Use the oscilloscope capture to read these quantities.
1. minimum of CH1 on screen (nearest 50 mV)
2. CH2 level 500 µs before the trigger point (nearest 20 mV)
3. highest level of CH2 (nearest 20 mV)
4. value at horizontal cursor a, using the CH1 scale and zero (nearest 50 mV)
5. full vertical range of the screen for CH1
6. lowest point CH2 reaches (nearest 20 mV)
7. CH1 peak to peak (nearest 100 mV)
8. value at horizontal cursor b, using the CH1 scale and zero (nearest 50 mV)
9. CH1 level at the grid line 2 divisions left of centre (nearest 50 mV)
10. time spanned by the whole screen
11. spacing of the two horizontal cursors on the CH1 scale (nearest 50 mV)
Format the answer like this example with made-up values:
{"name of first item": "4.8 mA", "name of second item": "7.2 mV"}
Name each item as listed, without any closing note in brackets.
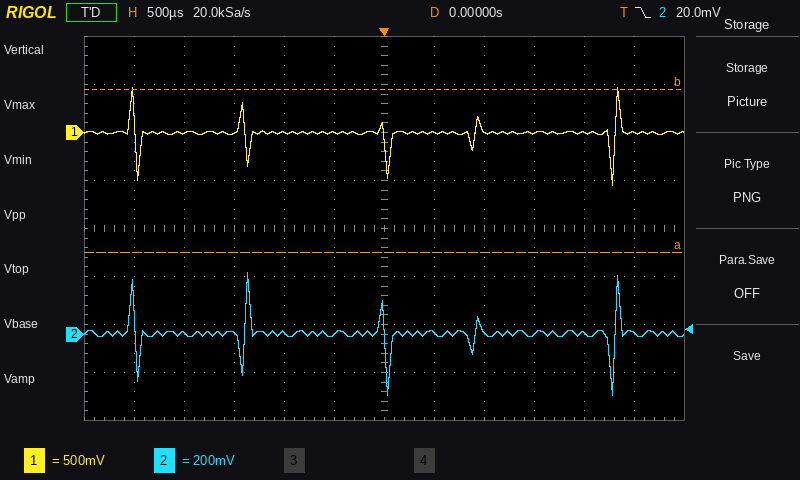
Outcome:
{"minimum of CH1 on screen": "-550 mV", "CH2 level 500 µs before the trigger point": "0 mV", "highest level of CH2": "260 mV", "value at horizontal cursor a, using the CH1 scale and zero": "-1.25 V", "full vertical range of the screen for CH1": "4 V", "lowest point CH2 reaches": "-260 mV", "CH1 peak to peak": "1.00 V", "value at horizontal cursor b, using the CH1 scale and zero": "450 mV", "CH1 level at the grid line 2 divisions left of centre": "0 mV", "time spanned by the whole screen": "6 ms", "spacing of the two horizontal cursors on the CH1 scale": "1.70 V"}
